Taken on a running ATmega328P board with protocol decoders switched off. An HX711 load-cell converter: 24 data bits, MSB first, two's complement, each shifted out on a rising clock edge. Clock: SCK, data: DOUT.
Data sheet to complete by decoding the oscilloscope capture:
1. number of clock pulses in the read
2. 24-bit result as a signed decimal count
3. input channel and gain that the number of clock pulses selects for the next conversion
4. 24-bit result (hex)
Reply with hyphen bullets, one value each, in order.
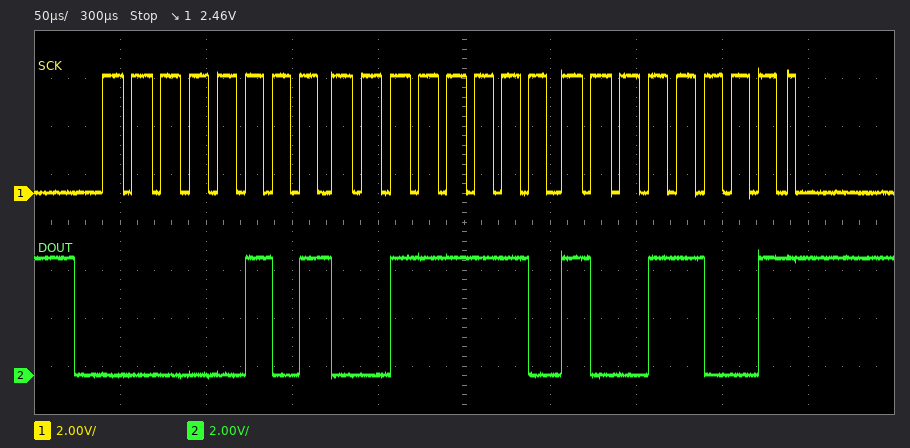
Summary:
- 25
- 343705
- channel A, gain 128
- 0x053E99
